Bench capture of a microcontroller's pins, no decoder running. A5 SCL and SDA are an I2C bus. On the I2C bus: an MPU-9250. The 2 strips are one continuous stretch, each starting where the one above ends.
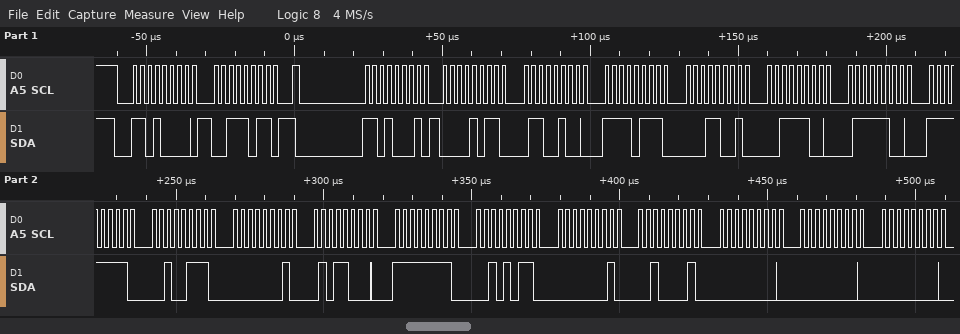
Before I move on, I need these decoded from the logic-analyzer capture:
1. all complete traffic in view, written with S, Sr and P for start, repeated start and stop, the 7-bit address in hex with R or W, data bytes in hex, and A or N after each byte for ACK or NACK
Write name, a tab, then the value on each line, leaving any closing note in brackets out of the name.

all complete traffic in view, written with S, Sr and P for start, repeated start and stop, the 7-bit address in hex with R or W, data bytes in hex, and A or N after each byte for ACK or NACK	S 68W A 3B A Sr 68R A 0B A 64 A F7 A 19 A 3C A 7C A FF A 27 A 01 A 58 A FF A 2B A 01 A 21 A 00 A 00 A 00 A
